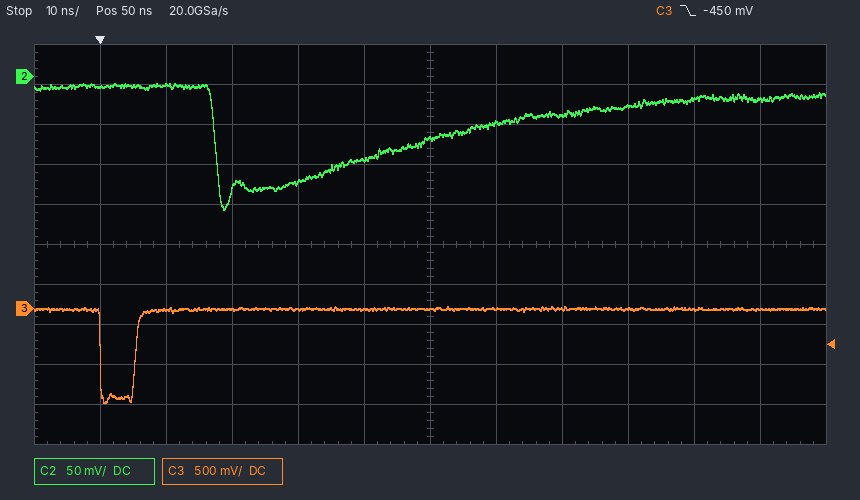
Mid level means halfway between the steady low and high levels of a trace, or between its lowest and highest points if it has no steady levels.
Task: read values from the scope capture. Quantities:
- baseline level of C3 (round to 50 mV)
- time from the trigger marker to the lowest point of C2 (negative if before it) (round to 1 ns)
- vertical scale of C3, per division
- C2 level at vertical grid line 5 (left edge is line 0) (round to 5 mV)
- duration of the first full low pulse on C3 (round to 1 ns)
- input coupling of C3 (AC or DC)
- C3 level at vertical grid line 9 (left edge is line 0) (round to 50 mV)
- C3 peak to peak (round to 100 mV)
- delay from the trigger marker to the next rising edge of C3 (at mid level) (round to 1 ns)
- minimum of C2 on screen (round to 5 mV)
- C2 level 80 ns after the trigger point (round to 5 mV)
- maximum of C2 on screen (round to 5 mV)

0 mV
+19 ns
500 mV
-105 mV
5 ns
DC
0 mV
1.20 V
5 ns
-165 mV
-35 mV
-10 mV
